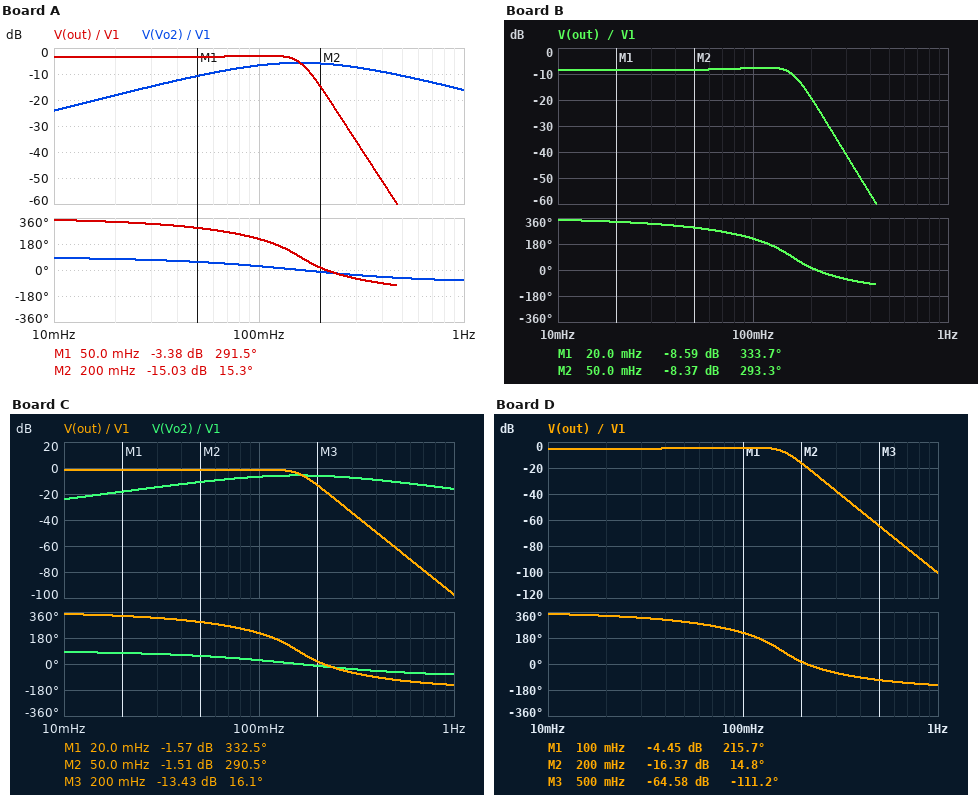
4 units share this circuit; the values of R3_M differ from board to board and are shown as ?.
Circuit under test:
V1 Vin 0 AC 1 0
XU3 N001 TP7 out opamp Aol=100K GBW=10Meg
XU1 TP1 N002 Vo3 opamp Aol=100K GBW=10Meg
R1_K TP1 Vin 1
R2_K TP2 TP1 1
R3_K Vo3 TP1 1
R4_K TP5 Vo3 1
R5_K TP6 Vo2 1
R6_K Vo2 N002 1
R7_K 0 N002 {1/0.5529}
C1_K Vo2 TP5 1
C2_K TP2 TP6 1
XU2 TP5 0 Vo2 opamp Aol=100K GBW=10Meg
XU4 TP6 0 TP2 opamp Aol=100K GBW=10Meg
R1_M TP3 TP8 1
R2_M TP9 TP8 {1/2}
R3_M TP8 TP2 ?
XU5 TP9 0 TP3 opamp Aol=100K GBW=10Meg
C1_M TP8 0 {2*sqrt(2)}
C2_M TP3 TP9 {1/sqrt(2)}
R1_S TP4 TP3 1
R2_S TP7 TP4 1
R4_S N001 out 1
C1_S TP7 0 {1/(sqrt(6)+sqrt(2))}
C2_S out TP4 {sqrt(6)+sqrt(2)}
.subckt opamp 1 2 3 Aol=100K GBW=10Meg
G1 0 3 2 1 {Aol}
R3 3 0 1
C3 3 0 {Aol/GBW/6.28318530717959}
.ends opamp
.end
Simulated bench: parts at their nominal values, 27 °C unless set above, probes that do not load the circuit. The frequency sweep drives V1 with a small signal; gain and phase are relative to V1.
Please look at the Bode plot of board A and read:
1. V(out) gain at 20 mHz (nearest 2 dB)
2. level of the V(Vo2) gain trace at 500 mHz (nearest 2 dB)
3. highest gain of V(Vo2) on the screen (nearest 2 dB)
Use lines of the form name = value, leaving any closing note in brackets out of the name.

V(out) gain at 20 mHz = -4 dB
level of the V(Vo2) gain trace at 500 mHz = -10 dB
highest gain of V(Vo2) on the screen = -6 dB
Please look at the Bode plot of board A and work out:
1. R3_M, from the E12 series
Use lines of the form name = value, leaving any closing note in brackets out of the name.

R3_M, from the E12 series = 1.5 Ω
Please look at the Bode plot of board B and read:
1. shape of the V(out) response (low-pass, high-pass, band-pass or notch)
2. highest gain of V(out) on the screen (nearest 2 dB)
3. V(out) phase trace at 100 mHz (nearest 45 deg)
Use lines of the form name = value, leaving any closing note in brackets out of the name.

shape of the V(out) response = low-pass
highest gain of V(out) on the screen = -8 dB
V(out) phase trace at 100 mHz = 225 deg
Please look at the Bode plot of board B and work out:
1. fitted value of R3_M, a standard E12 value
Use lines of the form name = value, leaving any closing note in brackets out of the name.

fitted value of R3_M, a standard E12 value = 2.7 Ω
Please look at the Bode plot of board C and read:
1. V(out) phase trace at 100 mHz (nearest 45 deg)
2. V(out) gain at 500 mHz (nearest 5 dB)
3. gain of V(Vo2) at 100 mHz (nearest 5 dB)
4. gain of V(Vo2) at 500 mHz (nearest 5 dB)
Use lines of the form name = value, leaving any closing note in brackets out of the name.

V(out) phase trace at 100 mHz = 225 deg
V(out) gain at 500 mHz = -60 dB
gain of V(Vo2) at 100 mHz = -5 dB
gain of V(Vo2) at 500 mHz = -10 dB
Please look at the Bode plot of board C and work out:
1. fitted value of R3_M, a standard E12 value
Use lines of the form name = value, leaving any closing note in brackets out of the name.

fitted value of R3_M, a standard E12 value = 1.2 Ω
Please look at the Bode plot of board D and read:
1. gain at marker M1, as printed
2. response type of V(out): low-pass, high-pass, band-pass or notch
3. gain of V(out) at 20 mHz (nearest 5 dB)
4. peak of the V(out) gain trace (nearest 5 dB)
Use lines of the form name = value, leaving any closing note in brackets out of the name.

gain at marker M1, as printed = -4.45 dB
response type of V(out): low-pass, high-pass, band-pass or notch = low-pass
gain of V(out) at 20 mHz = -5 dB
peak of the V(out) gain trace = -5 dB
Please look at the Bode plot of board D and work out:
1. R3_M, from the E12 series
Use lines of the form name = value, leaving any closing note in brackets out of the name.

R3_M, from the E12 series = 1.8 Ω
